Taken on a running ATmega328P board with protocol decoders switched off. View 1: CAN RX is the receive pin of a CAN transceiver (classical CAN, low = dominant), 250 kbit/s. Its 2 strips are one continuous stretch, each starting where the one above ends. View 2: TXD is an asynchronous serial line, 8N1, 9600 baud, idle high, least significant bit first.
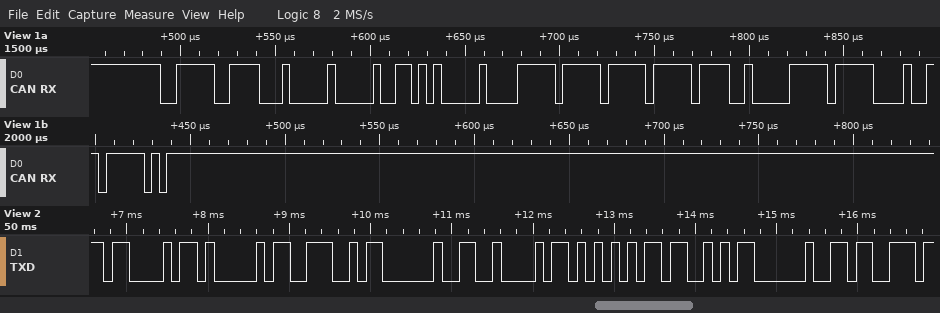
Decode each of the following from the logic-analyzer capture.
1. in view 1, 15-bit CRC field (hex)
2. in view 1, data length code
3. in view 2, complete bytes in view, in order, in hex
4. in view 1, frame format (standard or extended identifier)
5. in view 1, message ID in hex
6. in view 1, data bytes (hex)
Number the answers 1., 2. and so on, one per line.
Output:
1. 0x44DF
2. 8
3. 43 41 4E 20 42 55 53 20 73
4. standard
5. 0x3EF
6. 00 6A 00 FF FF FF 20 FF
